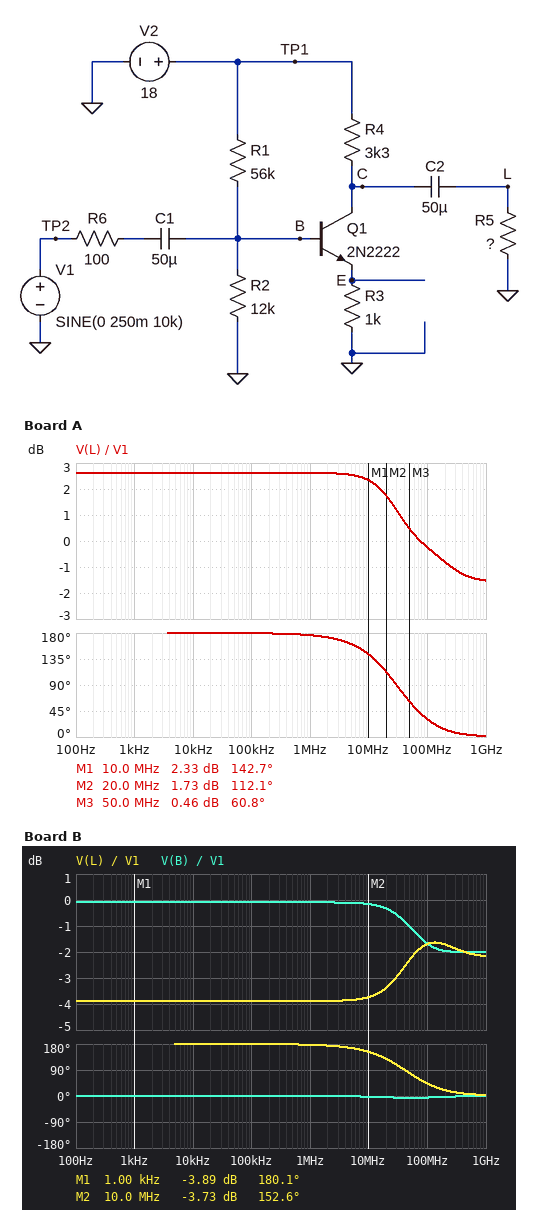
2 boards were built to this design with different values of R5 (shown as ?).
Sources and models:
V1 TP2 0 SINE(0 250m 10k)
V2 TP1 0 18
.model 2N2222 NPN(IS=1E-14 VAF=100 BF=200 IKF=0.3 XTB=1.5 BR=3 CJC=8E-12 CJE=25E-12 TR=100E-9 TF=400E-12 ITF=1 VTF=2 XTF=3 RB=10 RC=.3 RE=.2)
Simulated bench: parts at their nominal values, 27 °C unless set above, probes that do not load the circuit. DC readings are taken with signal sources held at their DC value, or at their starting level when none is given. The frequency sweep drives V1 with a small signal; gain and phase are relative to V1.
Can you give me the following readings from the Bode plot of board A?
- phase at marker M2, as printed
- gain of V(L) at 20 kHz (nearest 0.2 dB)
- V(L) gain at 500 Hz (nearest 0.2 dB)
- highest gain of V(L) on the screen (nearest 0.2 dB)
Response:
112.1 deg
2.6 dB
2.6 dB
2.6 dB
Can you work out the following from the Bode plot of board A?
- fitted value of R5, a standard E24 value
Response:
2.4 kΩ
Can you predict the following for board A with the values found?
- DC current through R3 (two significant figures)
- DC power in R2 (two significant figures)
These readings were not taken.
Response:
2.4 mA
780 µW
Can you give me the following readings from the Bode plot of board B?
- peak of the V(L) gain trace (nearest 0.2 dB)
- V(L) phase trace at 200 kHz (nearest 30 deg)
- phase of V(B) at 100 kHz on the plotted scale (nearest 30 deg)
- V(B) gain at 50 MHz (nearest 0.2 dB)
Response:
-1.6 dB
180 deg
0 deg
-1.0 dB
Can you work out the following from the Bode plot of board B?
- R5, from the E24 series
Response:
820 Ω
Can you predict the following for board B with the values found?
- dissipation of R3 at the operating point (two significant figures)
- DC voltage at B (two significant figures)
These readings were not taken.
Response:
5.7 mW
3.1 V
